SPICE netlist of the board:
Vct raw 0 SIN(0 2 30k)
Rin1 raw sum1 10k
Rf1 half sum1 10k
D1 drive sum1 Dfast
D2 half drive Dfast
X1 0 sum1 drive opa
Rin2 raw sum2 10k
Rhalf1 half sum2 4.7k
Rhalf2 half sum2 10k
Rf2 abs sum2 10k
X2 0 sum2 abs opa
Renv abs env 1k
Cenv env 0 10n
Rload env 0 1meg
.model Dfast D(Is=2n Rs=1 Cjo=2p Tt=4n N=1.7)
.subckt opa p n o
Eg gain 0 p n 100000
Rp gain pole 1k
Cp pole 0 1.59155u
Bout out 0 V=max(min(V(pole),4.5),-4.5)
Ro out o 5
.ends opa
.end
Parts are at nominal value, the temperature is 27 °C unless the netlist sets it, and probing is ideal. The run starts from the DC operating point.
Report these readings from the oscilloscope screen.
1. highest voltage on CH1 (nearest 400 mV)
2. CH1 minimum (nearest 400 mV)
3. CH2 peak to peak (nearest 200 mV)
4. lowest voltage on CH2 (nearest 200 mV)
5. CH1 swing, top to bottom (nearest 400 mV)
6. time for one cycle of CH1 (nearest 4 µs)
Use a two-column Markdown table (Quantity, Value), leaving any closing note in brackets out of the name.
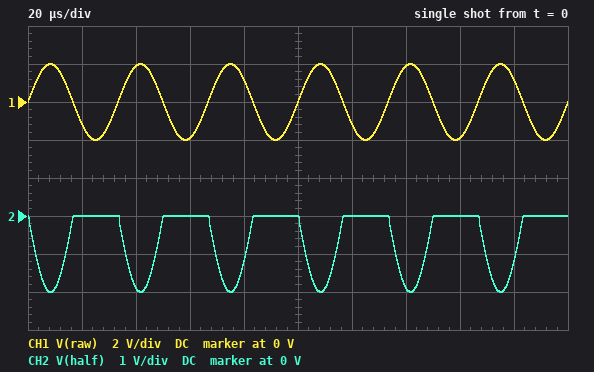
| Quantity | Value |
|---|---|
| highest voltage on CH1 | 2.0 V |
| CH1 minimum | -2.0 V |
| CH2 peak to peak | 2.0 V |
| lowest voltage on CH2 | -2.0 V |
| CH1 swing, top to bottom | 4.0 V |
| time for one cycle of CH1 | 32 µs |
